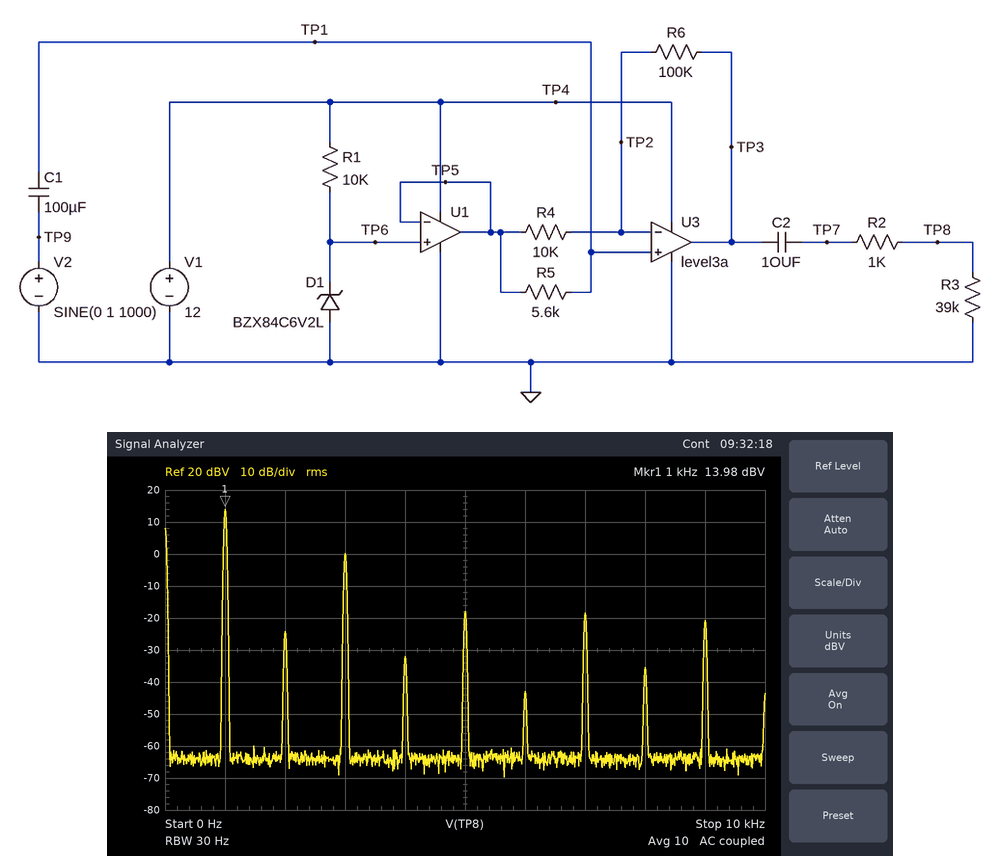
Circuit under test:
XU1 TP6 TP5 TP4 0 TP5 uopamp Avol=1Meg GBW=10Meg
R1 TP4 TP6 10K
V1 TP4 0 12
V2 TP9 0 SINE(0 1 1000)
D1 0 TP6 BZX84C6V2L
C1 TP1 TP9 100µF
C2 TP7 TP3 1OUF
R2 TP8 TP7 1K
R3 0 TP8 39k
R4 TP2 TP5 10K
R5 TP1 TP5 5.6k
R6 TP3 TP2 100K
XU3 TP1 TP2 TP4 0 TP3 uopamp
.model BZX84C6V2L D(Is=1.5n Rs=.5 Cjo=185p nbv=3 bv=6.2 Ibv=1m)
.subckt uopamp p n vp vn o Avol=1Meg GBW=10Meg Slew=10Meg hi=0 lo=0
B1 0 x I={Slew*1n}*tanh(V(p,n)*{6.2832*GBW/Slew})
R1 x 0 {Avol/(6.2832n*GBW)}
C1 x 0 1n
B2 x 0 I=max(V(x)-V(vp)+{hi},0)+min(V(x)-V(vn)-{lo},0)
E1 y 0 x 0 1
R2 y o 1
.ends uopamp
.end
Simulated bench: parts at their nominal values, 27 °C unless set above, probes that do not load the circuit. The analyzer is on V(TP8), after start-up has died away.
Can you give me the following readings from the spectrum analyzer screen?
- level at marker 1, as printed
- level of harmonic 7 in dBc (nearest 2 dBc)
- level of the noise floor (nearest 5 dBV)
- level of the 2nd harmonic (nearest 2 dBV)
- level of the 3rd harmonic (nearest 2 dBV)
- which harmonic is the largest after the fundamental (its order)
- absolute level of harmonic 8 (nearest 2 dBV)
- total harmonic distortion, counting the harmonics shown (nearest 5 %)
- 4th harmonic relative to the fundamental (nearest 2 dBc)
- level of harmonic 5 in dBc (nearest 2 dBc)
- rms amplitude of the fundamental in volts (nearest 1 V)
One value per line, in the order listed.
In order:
13.98 dBV
-32 dBc
-65 dBV
-24 dBV
0 dBV
3
-36 dBV
20 %
-46 dBc
-32 dBc
5 V
